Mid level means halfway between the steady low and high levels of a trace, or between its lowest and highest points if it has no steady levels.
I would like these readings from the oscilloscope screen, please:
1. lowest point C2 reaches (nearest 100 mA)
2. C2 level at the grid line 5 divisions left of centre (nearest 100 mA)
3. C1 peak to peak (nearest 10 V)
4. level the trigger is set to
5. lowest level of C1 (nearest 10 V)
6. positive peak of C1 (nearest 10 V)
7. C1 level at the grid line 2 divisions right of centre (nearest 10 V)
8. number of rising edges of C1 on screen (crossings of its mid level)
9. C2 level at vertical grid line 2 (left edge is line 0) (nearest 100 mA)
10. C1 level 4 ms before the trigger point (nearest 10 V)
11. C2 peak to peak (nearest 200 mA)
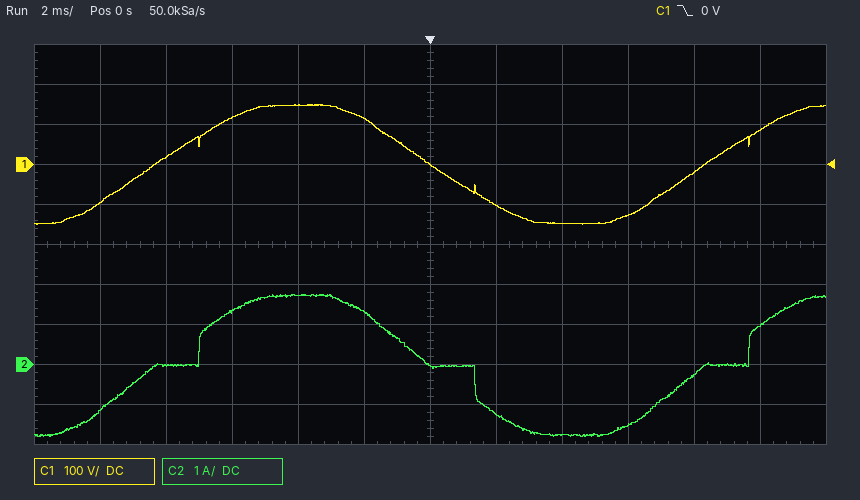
-1.8 A
-1.1 A
300 V
0 V
-150 V
150 V
-150 V
2
0.0 A
150 V
3.6 A
